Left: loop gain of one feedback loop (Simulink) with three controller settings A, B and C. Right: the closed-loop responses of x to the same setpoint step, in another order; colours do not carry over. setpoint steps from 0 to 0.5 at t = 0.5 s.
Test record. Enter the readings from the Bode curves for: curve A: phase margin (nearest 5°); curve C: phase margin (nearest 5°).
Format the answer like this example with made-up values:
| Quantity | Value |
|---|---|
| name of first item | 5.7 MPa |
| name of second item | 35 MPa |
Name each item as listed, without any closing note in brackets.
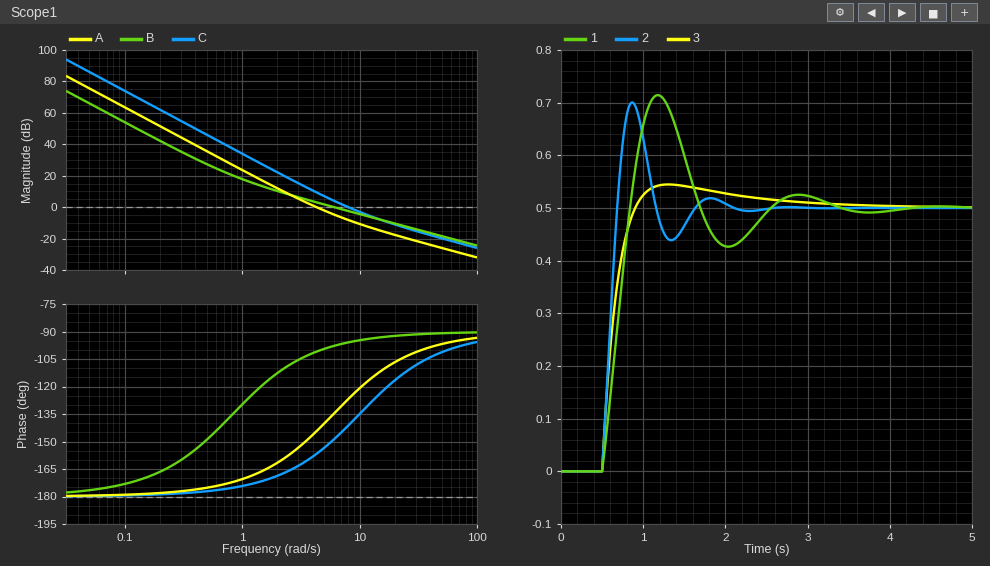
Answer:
| Quantity | Value |
|---|---|
| curve A: phase margin | 35° |
| curve C: phase margin | 40° |
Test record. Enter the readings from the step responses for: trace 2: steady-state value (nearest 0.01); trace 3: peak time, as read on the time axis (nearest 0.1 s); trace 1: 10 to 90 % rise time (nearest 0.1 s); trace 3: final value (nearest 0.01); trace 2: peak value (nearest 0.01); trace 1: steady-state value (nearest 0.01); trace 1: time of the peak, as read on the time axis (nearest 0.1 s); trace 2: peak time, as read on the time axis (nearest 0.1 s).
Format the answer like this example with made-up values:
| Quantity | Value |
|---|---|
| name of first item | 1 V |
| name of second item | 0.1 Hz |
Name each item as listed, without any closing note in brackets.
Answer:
| Quantity | Value |
|---|---|
| trace 2: steady-state value | 0.50 |
| trace 3: peak time, as read on the time axis | 1.3 s |
| trace 1: 10 to 90 % rise time | 0.3 s |
| trace 3: final value | 0.50 |
| trace 2: peak value | 0.70 |
| trace 1: steady-state value | 0.50 |
| trace 1: time of the peak, as read on the time axis | 1.2 s |
| trace 2: peak time, as read on the time axis | 0.9 s |
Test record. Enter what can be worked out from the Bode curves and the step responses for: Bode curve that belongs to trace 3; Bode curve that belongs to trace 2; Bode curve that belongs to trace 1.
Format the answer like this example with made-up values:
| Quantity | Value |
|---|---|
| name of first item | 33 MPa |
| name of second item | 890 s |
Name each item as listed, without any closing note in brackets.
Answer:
| Quantity | Value |
|---|---|
| Bode curve that belongs to trace 3 | B |
| Bode curve that belongs to trace 2 | C |
| Bode curve that belongs to trace 1 | A |
